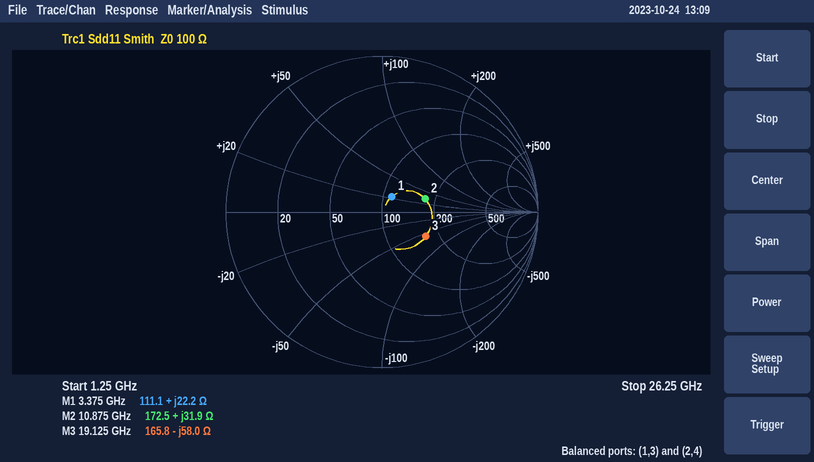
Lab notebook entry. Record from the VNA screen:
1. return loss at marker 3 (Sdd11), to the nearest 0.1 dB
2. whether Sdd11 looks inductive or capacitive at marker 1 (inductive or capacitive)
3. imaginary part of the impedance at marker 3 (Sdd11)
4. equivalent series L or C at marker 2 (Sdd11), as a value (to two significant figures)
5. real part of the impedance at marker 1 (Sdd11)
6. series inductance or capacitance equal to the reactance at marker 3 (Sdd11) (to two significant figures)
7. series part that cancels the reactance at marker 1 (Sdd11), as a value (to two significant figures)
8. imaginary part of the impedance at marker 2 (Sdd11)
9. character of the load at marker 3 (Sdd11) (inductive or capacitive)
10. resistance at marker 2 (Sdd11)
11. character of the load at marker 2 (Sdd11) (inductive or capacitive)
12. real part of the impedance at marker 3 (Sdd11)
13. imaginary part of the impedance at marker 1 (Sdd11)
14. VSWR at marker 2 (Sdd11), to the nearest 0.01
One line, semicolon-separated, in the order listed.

9.8 dB; inductive; -58.0 Ω; 470 pH; 111.1 Ω; 140 fF; 2.1 pF; +31.9 Ω; capacitive; 172.5 Ω; inductive; 165.8 Ω; +22.2 Ω; 1.81
